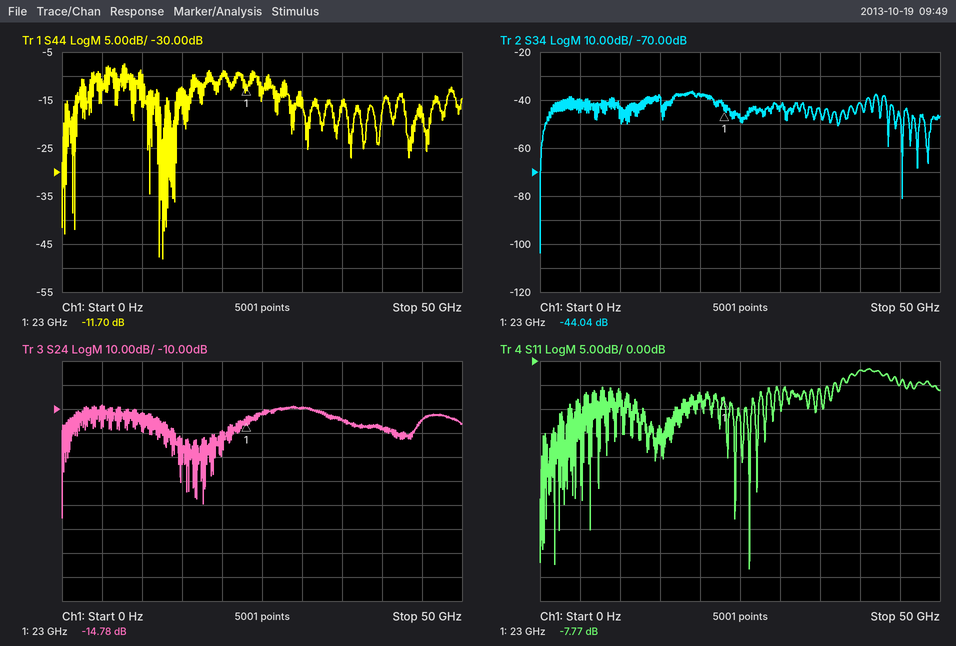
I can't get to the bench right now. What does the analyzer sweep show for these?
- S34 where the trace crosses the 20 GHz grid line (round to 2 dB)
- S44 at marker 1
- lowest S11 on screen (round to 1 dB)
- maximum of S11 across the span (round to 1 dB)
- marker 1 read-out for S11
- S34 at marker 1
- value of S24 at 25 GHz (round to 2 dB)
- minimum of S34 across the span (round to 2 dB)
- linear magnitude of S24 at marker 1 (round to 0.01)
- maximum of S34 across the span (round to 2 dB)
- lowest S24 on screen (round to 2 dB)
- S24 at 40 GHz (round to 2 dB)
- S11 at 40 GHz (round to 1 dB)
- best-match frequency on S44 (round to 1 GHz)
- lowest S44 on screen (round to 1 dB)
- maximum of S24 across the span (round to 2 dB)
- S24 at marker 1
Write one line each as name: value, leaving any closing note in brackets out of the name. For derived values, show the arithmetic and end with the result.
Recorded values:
S34 where the trace crosses the 20 GHz grid line: -38 dB
S44 at marker 1: -11.70 dB
lowest S11 on screen: -43 dB
maximum of S11 across the span: -2 dB
marker 1 read-out for S11: -7.77 dB
S34 at marker 1: -44.04 dB
value of S24 at 25 GHz: -12 dB
minimum of S34 across the span: -104 dB
linear magnitude of S24 at marker 1: 10^(-14.78/20) ≈ 0.18
maximum of S34 across the span: -36 dB
lowest S24 on screen: -56 dB
S24 at 40 GHz: -18 dB
S11 at 40 GHz: -2 dB
best-match frequency on S44: 13 GHz
lowest S44 on screen: -48 dB
maximum of S24 across the span: -8 dB
S24 at marker 1: -14.78 dB
